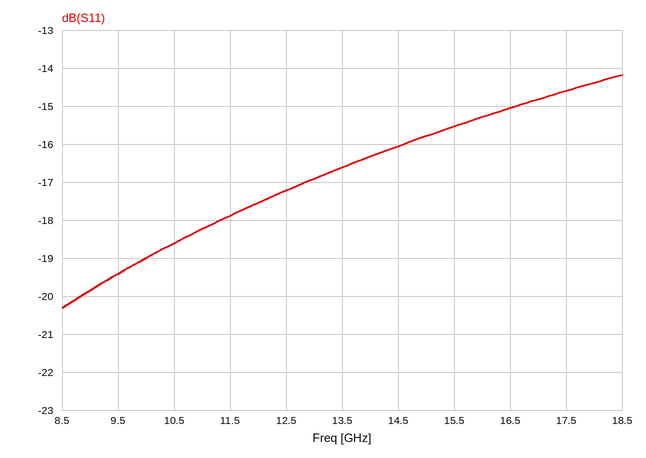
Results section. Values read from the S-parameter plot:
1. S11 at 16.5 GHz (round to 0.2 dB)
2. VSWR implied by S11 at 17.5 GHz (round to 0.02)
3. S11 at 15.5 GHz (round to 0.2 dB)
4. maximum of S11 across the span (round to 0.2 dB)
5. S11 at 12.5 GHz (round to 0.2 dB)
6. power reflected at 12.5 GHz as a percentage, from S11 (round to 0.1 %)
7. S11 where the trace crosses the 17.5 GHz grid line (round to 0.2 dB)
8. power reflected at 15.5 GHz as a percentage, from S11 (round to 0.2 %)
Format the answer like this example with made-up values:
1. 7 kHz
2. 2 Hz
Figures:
1. -15.0 dB
2. 1.46
3. -15.6 dB
4. -14.2 dB
5. -17.2 dB
6. 1.9 %
7. -14.6 dB
8. 2.8 %
